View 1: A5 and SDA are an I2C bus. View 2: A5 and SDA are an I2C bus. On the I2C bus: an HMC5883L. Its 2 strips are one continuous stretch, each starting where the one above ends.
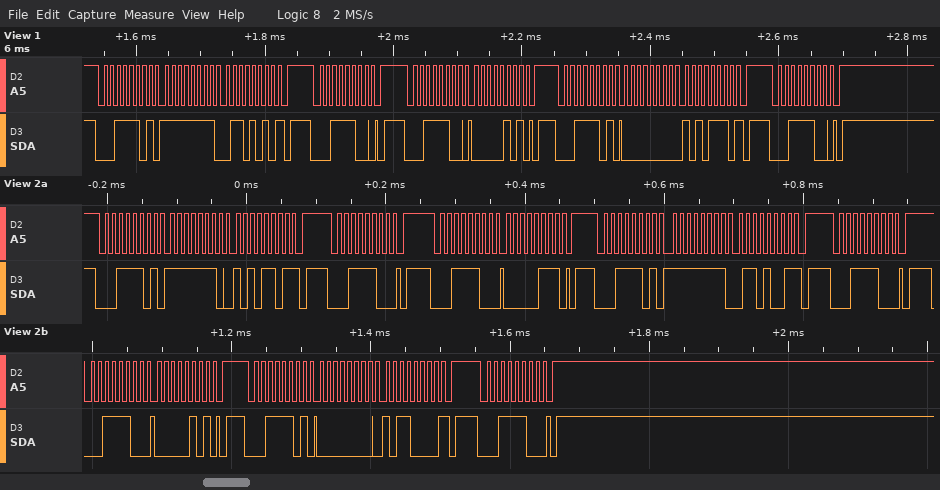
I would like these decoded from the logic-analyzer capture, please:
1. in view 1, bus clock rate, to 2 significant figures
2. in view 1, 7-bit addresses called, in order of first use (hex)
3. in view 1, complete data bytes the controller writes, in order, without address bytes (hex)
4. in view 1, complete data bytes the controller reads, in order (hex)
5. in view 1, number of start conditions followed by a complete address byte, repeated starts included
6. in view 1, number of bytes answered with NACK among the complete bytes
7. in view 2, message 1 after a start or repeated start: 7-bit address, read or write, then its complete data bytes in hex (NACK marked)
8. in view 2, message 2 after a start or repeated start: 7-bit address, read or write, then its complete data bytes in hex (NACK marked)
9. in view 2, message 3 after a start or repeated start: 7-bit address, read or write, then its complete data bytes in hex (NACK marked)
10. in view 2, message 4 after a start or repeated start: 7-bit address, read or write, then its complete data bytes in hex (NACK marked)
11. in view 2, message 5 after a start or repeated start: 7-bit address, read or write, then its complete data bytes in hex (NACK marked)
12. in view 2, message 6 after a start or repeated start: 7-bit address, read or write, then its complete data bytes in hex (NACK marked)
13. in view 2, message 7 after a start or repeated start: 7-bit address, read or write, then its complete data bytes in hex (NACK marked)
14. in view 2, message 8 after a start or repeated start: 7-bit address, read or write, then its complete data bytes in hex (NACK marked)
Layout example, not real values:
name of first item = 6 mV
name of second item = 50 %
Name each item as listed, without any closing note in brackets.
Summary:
in view 1, bus clock rate, to 2 significant figures = 100 kHz
in view 1, 7-bit addresses called, in order of first use = 0x1E
in view 1, complete data bytes the controller writes, in order, without address bytes = 05
in view 1, complete data bytes the controller reads, in order = FF 6A 00 AE
in view 1, number of start conditions followed by a complete address byte, repeated starts included = 5
in view 1, number of bytes answered with NACK among the complete bytes = 2
in view 2, message 1 after a start or repeated start: 7-bit address, read or write, then its complete data bytes in hex = 0x1E read: FE AD NACK
in view 2, message 2 after a start or repeated start: 7-bit address, read or write, then its complete data bytes in hex = 0x1E write
in view 2, message 3 after a start or repeated start: 7-bit address, read or write, then its complete data bytes in hex = 0x1E write: 07
in view 2, message 4 after a start or repeated start: 7-bit address, read or write, then its complete data bytes in hex = 0x1E read: FF 69 NACK
in view 2, message 5 after a start or repeated start: 7-bit address, read or write, then its complete data bytes in hex = 0x1E write
in view 2, message 6 after a start or repeated start: 7-bit address, read or write, then its complete data bytes in hex = 0x1E write: 05
in view 2, message 7 after a start or repeated start: 7-bit address, read or write, then its complete data bytes in hex = 0x1E read: 00 B0 NACK
in view 2, message 8 after a start or repeated start: 7-bit address, read or write, then its complete data bytes in hex = 0x1E write
